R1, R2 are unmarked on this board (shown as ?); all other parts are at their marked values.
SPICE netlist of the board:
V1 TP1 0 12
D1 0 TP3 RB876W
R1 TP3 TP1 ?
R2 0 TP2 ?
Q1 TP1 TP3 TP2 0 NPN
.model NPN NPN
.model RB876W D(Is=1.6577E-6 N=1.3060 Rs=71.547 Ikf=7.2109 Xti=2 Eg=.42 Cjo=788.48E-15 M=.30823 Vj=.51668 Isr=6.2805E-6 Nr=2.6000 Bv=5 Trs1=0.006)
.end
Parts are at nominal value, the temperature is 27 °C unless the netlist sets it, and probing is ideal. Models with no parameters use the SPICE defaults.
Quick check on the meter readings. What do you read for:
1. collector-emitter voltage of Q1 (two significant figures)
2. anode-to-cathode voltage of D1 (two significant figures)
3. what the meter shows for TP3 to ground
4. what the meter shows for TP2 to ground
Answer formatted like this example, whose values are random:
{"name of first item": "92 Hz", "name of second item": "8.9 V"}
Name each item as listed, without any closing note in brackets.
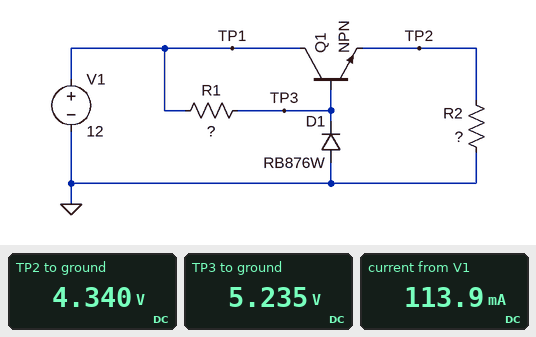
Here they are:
{"collector-emitter voltage of Q1": "7.7 V", "anode-to-cathode voltage of D1": "-5.2 V", "what the meter shows for TP3 to ground": "5.235 V", "what the meter shows for TP2 to ground": "4.340 V"}
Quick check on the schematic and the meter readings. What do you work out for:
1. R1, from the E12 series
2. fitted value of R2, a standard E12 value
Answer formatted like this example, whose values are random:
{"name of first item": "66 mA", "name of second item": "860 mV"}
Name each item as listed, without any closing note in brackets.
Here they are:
{"R1, from the E12 series": "1.8 kΩ", "fitted value of R2, a standard E12 value": "39 Ω"}
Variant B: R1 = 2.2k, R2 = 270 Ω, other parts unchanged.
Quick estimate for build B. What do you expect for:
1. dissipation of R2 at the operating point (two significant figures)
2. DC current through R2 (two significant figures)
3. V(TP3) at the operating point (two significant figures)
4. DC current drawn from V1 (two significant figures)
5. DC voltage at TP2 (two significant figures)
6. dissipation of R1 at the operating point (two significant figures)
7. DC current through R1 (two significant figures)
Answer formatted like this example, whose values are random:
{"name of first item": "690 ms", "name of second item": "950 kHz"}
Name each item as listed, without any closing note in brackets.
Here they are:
{"dissipation of R2 at the operating point": "72 mW", "DC current through R2": "16 mA", "V(TP3) at the operating point": "5.3 V", "DC current drawn from V1": "19 mA", "DC voltage at TP2": "4.4 V", "dissipation of R1 at the operating point": "21 mW", "DC current through R1": "3.1 mA"}
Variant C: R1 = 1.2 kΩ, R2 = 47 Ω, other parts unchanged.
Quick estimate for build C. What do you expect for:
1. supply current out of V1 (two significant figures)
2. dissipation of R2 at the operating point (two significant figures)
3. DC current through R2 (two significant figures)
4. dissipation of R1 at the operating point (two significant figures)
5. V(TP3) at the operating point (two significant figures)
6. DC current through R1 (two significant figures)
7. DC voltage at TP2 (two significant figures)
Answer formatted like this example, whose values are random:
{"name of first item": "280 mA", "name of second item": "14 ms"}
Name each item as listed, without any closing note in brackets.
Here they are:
{"supply current out of V1": "100 mA", "dissipation of R2 at the operating point": "430 mW", "DC current through R2": "96 mA", "dissipation of R1 at the operating point": "36 mW", "V(TP3) at the operating point": "5.4 V", "DC current through R1": "5.5 mA", "DC voltage at TP2": "4.5 V"}
